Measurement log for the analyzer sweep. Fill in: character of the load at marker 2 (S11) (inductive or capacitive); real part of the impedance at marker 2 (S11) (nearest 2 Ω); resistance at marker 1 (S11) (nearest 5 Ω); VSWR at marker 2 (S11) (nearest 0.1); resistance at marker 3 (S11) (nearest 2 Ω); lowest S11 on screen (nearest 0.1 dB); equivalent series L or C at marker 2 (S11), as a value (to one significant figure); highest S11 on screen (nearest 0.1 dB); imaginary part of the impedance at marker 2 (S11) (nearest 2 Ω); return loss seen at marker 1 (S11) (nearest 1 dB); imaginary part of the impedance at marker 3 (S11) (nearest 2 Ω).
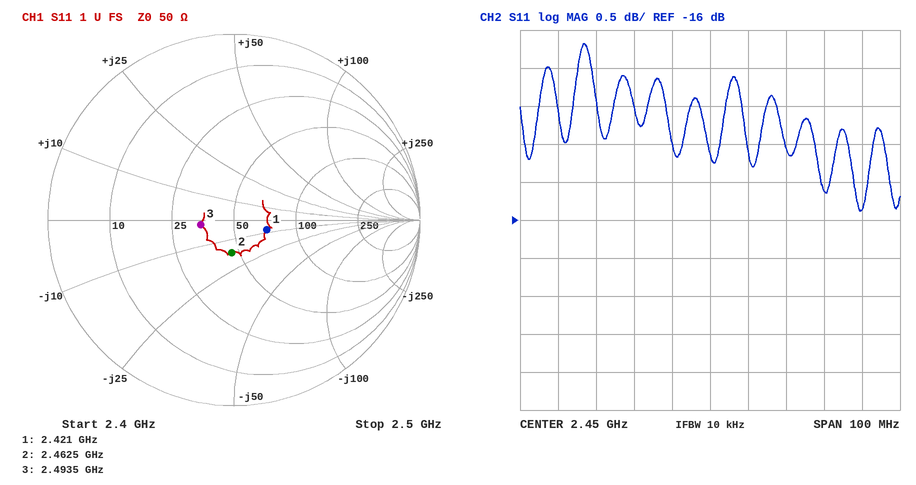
capacitive
46 Ω
70 Ω
1.4
34 Ω
-15.9 dB
4 pF
-13.7 dB
-16 Ω
15 dB
-2 Ω
